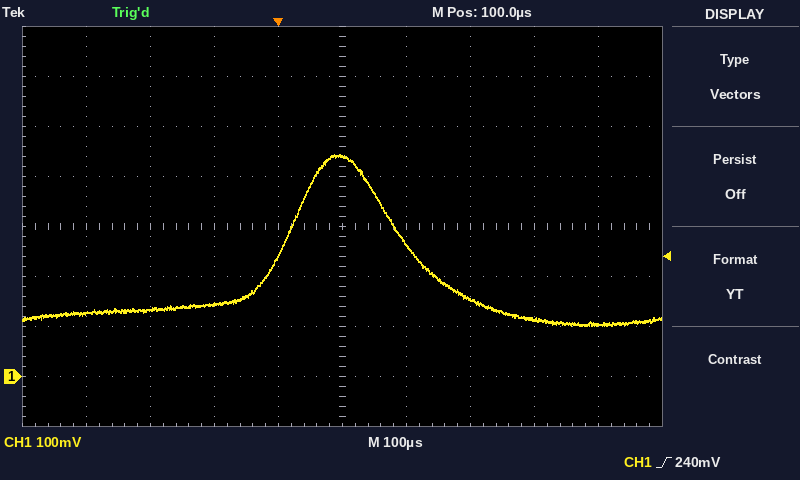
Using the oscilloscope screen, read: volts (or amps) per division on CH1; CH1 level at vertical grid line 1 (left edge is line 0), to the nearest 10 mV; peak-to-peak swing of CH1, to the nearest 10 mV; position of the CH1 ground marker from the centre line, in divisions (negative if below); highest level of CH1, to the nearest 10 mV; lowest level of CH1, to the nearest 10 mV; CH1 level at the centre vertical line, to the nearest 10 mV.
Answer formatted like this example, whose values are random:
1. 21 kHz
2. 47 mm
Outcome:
1. 100 mV
2. 130 mV
3. 340 mV
4. -3.0 div
5. 440 mV
6. 100 mV
7. 440 mV
